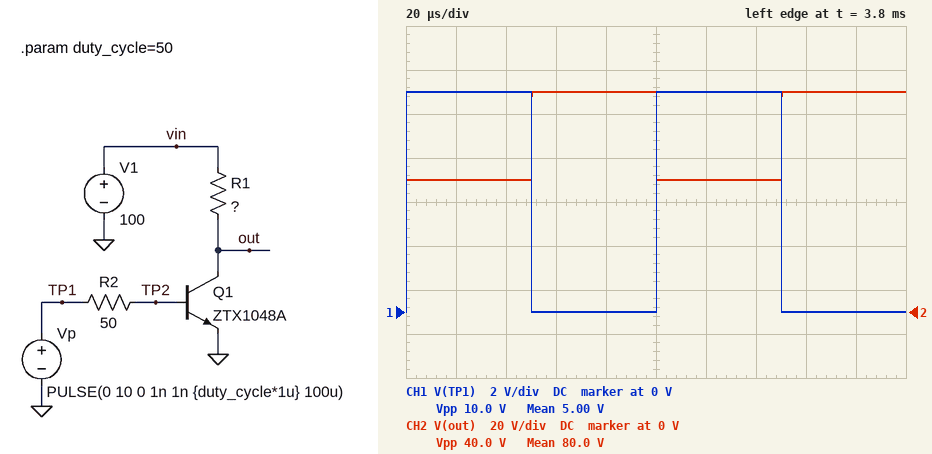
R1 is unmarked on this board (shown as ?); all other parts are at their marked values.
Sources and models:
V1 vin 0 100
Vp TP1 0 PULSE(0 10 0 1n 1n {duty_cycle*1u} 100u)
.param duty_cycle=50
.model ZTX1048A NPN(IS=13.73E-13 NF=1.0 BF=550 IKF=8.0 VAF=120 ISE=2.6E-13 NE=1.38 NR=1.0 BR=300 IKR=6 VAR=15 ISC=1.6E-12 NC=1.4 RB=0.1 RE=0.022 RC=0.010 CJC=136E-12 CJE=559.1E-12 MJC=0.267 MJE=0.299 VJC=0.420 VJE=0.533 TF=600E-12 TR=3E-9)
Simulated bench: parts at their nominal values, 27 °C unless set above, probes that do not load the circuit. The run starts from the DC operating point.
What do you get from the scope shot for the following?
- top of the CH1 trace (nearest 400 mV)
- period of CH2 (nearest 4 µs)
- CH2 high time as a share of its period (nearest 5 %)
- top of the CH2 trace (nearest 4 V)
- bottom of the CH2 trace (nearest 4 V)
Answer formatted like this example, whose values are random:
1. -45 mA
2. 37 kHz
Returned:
1. 10.0 V
2. 100 µs
3. 50 %
4. 100 V
5. 60 V
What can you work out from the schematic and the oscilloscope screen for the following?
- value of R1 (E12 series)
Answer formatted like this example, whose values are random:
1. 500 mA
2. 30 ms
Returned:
1. 1.2 Ω
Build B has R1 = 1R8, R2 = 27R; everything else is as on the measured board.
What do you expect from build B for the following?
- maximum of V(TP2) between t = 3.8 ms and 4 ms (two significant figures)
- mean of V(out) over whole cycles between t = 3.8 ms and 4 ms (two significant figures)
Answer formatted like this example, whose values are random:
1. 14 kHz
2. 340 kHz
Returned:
1. 1.7 V
2. 65 V
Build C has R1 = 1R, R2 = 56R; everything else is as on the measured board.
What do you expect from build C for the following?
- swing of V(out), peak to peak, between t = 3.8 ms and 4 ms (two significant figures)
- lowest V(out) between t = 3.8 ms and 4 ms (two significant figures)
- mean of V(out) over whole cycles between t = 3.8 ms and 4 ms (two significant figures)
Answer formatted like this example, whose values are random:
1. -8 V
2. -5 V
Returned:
1. 33 V
2. 67 V
3. 84 V
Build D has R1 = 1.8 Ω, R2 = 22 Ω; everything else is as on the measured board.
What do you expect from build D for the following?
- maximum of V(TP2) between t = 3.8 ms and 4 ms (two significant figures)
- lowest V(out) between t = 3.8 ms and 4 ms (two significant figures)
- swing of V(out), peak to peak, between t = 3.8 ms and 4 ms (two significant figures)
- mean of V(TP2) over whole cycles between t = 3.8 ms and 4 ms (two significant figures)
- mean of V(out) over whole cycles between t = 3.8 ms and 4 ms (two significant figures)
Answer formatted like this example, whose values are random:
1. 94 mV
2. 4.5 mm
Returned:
1. 1.8 V
2. 25 V
3. 75 V
4. 900 mV
5. 63 V
